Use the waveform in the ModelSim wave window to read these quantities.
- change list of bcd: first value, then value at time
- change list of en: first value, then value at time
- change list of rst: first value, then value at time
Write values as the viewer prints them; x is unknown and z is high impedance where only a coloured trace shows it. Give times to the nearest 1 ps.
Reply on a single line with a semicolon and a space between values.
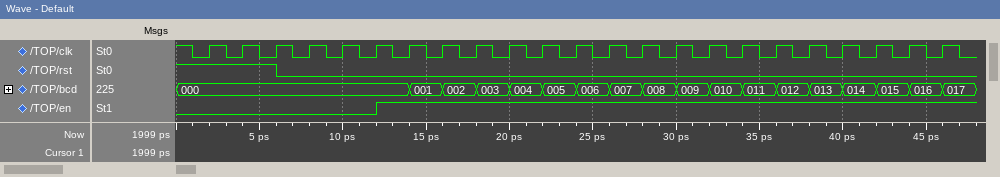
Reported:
000, 001 at 14 ps, 002 at 16 ps, 003 at 18 ps, 004 at 20 ps, 005 at 22 ps, 006 at 24 ps, 007 at 26 ps, 008 at 28 ps, 009 at 30 ps, 010 at 32 ps, 011 at 34 ps, 012 at 36 ps, 013 at 38 ps, 014 at 40 ps, 015 at 42 ps, 016 at 44 ps, 017 at 46 ps; 0, 1 at 12 ps; 1, 0 at 6 ps
